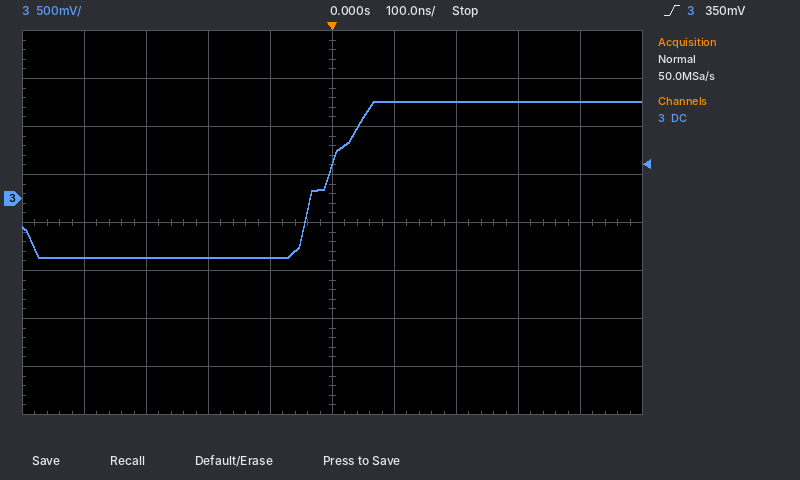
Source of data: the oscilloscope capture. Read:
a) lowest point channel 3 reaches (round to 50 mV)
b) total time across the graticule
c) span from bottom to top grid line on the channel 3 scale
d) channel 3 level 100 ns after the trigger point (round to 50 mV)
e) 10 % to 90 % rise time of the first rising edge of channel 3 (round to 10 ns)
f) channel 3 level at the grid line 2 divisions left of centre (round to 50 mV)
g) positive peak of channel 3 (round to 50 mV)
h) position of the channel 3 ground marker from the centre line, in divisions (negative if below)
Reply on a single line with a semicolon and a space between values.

-600 mV; 1 µs; 4 V; 1.00 V; 100 ns; -600 mV; 1.00 V; +0.5 div
